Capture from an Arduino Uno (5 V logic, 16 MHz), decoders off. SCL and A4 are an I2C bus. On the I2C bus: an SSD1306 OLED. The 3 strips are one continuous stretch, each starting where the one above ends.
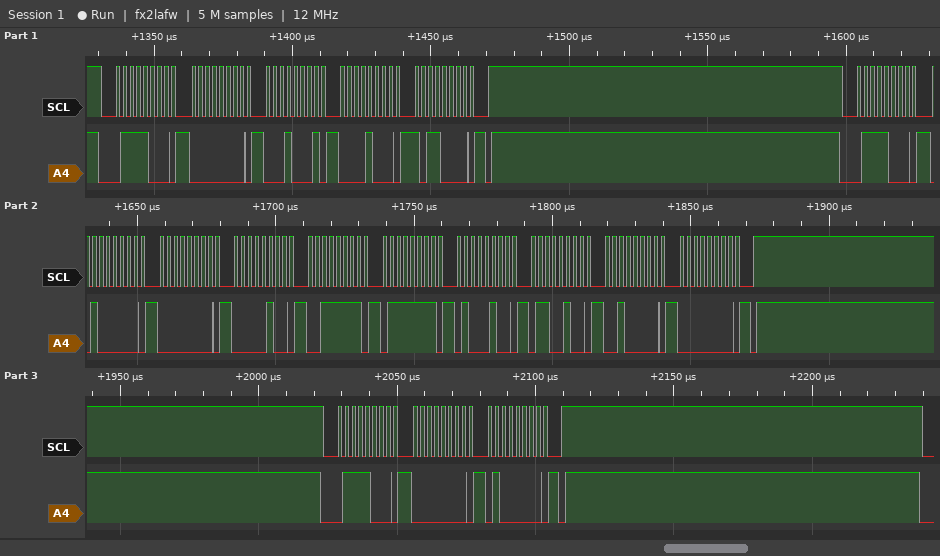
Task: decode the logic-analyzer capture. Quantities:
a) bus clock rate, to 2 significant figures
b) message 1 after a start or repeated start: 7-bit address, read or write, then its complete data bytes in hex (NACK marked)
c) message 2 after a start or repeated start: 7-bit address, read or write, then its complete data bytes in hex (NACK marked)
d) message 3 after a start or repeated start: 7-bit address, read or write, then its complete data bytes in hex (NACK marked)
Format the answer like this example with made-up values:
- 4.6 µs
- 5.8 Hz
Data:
- 400 kHz
- 0x3C write: 00 11 08 B0
- 0x3C write: 40 00 04 3F 7F 44 64 20 00
- 0x3C write: 00 40
